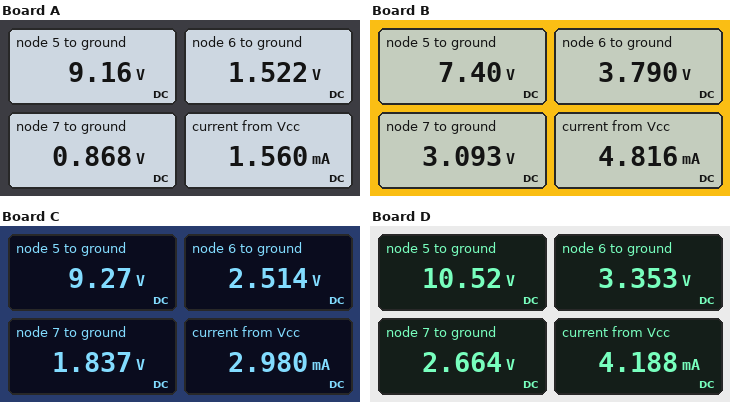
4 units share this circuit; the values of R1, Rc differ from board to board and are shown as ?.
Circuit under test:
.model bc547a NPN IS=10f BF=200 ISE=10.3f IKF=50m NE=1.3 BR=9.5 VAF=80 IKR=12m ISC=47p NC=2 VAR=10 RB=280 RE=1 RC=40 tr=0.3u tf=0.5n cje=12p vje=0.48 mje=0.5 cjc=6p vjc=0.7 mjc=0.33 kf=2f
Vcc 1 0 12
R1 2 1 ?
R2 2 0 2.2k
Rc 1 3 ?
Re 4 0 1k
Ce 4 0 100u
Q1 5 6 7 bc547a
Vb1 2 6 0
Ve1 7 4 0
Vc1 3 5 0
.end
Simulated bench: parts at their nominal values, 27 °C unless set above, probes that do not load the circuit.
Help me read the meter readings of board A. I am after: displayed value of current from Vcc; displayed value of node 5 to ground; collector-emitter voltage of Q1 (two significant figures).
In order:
1.560 mA
9.16 V
8.3 V
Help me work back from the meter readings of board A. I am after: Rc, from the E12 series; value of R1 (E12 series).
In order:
3.3 kΩ
15 kΩ
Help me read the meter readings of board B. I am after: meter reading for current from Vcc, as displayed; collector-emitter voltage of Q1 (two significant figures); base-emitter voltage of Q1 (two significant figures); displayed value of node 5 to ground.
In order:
4.816 mA
4.3 V
700 mV
7.40 V
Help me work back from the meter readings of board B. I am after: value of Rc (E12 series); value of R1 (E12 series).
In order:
1.5 kΩ
4.7 kΩ
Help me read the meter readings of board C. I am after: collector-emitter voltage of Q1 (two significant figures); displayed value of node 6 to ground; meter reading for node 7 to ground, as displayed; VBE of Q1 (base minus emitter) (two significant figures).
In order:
7.4 V
2.514 V
1.837 V
680 mV
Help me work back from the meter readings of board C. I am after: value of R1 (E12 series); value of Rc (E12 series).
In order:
8.2 kΩ
1.5 kΩ
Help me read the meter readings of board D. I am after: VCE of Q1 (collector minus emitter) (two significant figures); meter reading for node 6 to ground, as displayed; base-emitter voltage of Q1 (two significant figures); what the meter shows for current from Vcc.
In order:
7.9 V
3.353 V
690 mV
4.188 mA
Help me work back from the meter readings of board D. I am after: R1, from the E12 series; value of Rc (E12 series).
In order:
5.6 kΩ
560 Ω
